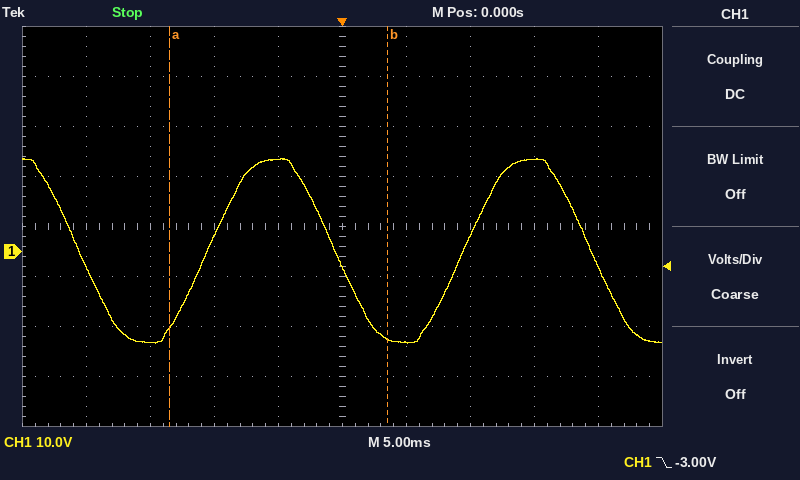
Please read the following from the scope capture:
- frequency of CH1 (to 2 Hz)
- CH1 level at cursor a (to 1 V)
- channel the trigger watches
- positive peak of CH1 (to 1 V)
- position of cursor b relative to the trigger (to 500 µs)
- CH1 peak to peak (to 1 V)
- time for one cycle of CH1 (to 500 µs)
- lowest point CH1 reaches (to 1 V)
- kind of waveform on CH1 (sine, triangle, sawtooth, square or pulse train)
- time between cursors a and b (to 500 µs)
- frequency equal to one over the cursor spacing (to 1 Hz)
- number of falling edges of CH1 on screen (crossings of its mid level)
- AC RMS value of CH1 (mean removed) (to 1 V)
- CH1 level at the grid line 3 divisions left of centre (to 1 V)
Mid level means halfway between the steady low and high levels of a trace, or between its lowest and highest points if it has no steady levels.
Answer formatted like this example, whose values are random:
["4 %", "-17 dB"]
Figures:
["50 Hz", "-15 V", "CH1", "19 V", "+3.5 ms", "37 V", "20.0 ms", "-18 V", "sine", "17.0 ms", "59 Hz", "3", "13 V", "-18 V"]
